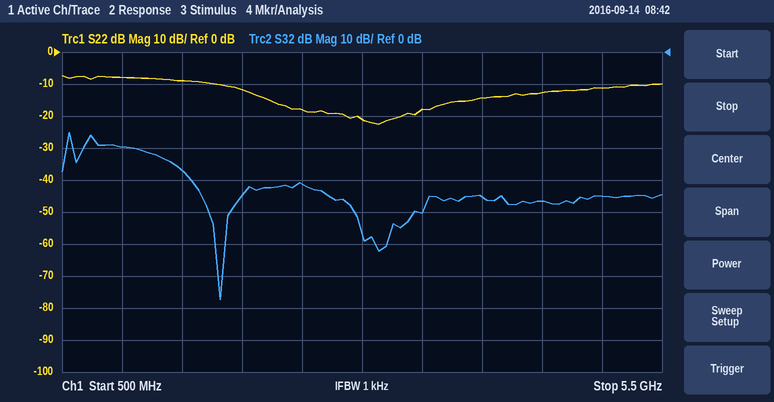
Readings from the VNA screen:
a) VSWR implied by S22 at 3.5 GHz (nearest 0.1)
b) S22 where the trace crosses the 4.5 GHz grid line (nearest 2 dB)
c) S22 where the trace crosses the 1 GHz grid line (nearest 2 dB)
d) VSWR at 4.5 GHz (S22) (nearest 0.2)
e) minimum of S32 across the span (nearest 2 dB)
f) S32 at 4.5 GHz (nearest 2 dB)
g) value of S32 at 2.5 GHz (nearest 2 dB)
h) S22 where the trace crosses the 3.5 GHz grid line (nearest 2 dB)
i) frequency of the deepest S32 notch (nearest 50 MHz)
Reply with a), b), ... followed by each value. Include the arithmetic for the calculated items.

a) |Γ| = 10^(-18/20) = 0.1259; VSWR = (1 + 0.1259)/(1 − 0.1259) ≈ 1.3
b) -12 dB
c) -8 dB
d) |Γ| = 10^(-12/20) = 0.2512; VSWR = (1 + 0.2512)/(1 − 0.2512) ≈ 1.67, so 1.6 to the nearest 0.2
e) -78 dB
f) -46 dB
g) -42 dB
h) -18 dB
i) 1.80 GHz
